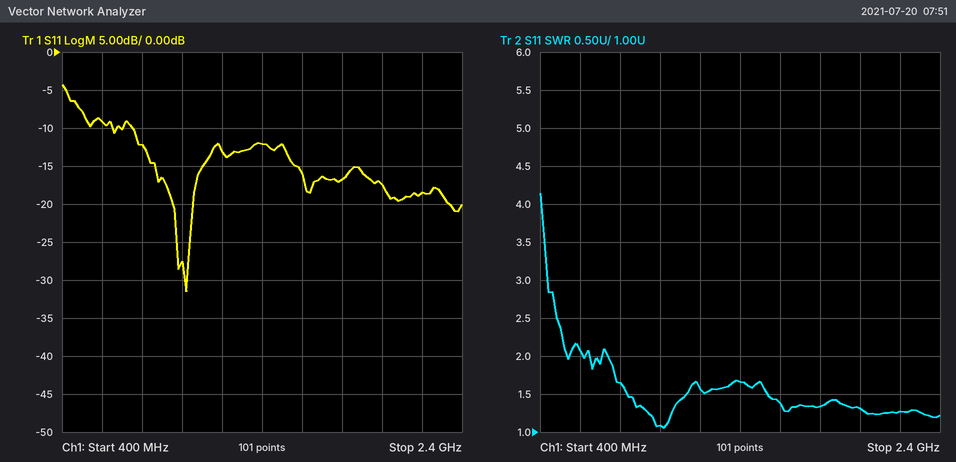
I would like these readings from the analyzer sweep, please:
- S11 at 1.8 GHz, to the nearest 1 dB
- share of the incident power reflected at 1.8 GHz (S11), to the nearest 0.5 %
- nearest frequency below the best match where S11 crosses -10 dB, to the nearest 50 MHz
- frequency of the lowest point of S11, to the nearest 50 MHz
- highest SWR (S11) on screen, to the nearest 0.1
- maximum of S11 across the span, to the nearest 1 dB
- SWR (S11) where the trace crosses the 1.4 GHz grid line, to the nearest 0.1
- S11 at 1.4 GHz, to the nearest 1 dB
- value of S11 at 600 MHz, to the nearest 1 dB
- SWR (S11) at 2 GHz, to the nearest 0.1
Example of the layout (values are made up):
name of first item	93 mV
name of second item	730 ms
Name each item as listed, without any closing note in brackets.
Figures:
S11 at 1.8 GHz, to the nearest 1 dB	-17 dB
share of the incident power reflected at 1.8 GHz (S11), to the nearest 0.5 %	2.0 %
nearest frequency below the best match where S11 crosses -10 dB, to the nearest 50 MHz	750 MHz
frequency of the lowest point of S11, to the nearest 50 MHz	1.00 GHz
highest SWR (S11) on screen, to the nearest 0.1	4.1
maximum of S11 across the span, to the nearest 1 dB	-4 dB
SWR (S11) where the trace crosses the 1.4 GHz grid line, to the nearest 0.1	1.7
S11 at 1.4 GHz, to the nearest 1 dB	-12 dB
value of S11 at 600 MHz, to the nearest 1 dB	-9 dB
SWR (S11) at 2 GHz, to the nearest 0.1	1.3
